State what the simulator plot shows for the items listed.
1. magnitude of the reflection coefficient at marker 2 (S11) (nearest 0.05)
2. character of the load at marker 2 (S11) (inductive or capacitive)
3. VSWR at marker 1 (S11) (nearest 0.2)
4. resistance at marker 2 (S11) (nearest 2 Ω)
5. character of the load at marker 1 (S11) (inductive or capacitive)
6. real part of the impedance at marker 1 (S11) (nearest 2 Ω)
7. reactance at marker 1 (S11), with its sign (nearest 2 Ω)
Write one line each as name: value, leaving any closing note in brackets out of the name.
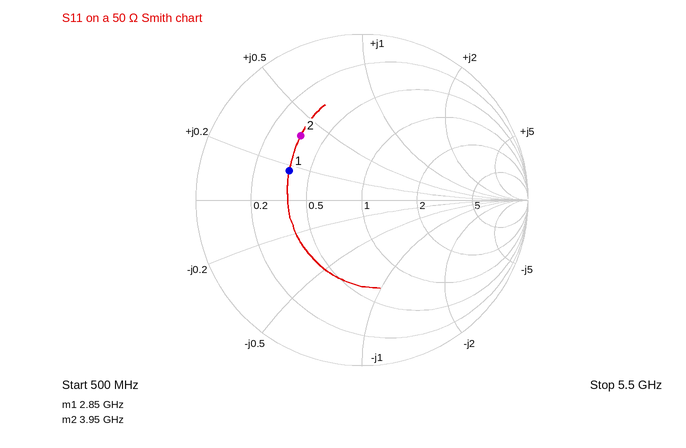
magnitude of the reflection coefficient at marker 2 (S11): 0.55
character of the load at marker 2 (S11): inductive
VSWR at marker 1 (S11): 2.8
resistance at marker 2 (S11): 18 Ω
character of the load at marker 1 (S11): inductive
real part of the impedance at marker 1 (S11): 18 Ω
reactance at marker 1 (S11), with its sign: +8 Ω
